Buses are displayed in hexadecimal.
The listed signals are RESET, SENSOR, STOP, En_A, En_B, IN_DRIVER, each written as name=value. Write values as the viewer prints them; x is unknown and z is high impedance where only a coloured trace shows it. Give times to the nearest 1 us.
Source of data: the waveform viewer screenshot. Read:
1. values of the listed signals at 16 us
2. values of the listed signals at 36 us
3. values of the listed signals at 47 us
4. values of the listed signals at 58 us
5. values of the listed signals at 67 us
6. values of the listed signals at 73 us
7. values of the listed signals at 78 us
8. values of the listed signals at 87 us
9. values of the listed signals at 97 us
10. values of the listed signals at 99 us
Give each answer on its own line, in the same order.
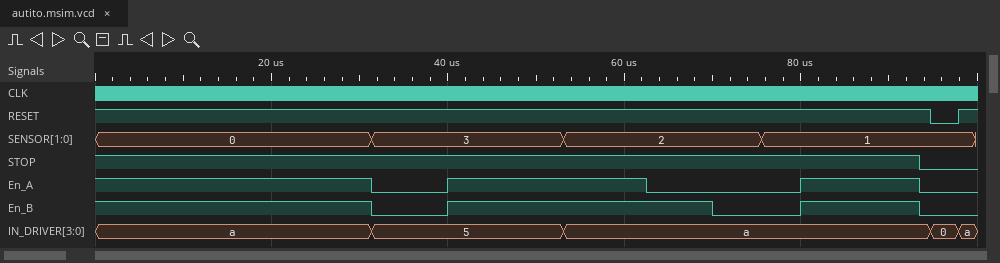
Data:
RESET=1, SENSOR=0, STOP=1, En_A=1, En_B=1, IN_DRIVER=a
RESET=1, SENSOR=3, STOP=1, En_A=0, En_B=0, IN_DRIVER=5
RESET=1, SENSOR=3, STOP=1, En_A=1, En_B=1, IN_DRIVER=5
RESET=1, SENSOR=2, STOP=1, En_A=1, En_B=1, IN_DRIVER=a
RESET=1, SENSOR=2, STOP=1, En_A=0, En_B=1, IN_DRIVER=a
RESET=1, SENSOR=2, STOP=1, En_A=0, En_B=0, IN_DRIVER=a
RESET=1, SENSOR=1, STOP=1, En_A=0, En_B=0, IN_DRIVER=a
RESET=1, SENSOR=1, STOP=1, En_A=1, En_B=1, IN_DRIVER=a
RESET=0, SENSOR=1, STOP=0, En_A=0, En_B=0, IN_DRIVER=0
RESET=1, SENSOR=1, STOP=0, En_A=0, En_B=0, IN_DRIVER=a
